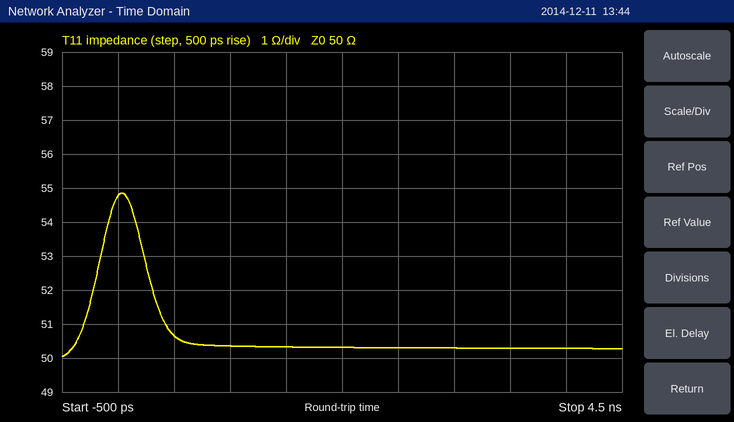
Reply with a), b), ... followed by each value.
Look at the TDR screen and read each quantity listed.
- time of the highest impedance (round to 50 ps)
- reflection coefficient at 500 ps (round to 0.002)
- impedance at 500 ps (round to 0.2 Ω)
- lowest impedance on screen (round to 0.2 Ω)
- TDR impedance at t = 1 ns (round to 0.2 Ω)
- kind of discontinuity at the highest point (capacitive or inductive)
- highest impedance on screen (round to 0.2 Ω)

a) 50 ps
b) +0.006
c) 50.6 Ω
d) 50.0 Ω
e) 50.4 Ω
f) inductive
g) 54.8 Ω
